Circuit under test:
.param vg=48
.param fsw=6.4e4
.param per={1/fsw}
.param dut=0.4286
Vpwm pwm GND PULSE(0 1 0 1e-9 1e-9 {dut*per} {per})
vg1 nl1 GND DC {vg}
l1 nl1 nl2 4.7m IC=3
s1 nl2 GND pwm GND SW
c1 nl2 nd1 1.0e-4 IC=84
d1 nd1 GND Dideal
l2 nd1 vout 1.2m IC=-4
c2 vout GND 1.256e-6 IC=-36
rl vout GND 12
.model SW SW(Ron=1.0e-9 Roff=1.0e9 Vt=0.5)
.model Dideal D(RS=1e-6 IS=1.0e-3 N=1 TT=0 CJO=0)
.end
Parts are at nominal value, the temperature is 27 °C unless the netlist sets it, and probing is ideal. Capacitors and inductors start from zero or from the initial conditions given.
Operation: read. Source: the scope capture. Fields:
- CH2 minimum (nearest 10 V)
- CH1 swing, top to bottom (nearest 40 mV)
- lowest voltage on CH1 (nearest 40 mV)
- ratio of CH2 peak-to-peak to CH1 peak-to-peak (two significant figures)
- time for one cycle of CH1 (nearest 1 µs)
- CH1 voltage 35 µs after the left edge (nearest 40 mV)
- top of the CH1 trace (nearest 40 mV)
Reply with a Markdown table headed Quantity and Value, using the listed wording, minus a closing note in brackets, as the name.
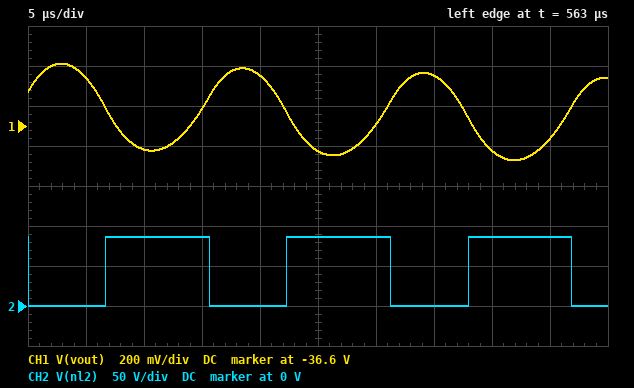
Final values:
| Quantity | Value |
|---|---|
| CH2 minimum | 0 V |
| CH1 swing, top to bottom | 480 mV |
| lowest voltage on CH1 | -36.76 V |
| ratio of CH2 peak-to-peak to CH1 peak-to-peak | 180 |
| time for one cycle of CH1 | 16 µs |
| CH1 voltage 35 µs after the left edge | -36.36 V |
| top of the CH1 trace | -36.28 V |
